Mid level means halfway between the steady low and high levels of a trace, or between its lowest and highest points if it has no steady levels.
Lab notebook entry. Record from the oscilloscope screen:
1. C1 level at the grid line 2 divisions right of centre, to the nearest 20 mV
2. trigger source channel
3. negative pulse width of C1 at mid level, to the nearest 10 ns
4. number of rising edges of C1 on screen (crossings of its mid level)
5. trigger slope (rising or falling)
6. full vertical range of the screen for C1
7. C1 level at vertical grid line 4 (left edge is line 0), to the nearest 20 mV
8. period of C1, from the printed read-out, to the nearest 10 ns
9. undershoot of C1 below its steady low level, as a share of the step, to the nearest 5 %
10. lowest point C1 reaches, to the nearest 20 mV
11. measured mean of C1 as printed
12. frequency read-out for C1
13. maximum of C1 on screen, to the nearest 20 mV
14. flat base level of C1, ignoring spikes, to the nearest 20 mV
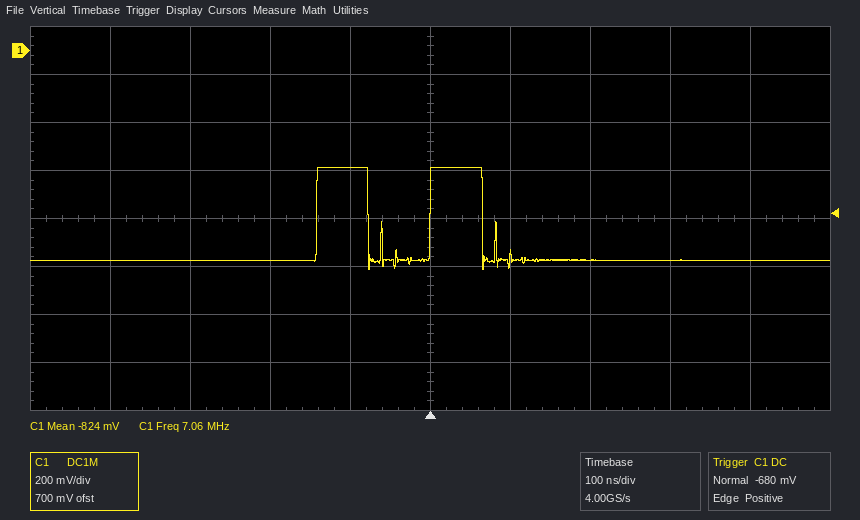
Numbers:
-880 mV
C1
80 ns
2
rising
1.6 V
-480 mV
140 ns
10 %
-920 mV
-824 mV
7.06 MHz
-480 mV
-880 mV
